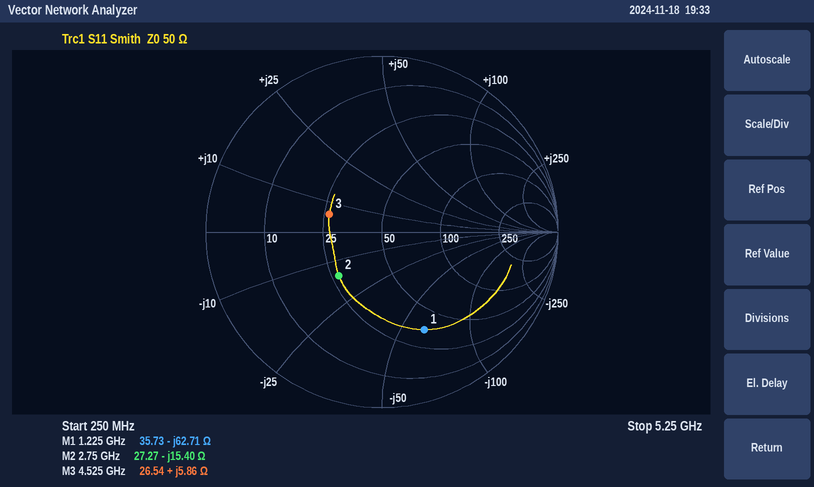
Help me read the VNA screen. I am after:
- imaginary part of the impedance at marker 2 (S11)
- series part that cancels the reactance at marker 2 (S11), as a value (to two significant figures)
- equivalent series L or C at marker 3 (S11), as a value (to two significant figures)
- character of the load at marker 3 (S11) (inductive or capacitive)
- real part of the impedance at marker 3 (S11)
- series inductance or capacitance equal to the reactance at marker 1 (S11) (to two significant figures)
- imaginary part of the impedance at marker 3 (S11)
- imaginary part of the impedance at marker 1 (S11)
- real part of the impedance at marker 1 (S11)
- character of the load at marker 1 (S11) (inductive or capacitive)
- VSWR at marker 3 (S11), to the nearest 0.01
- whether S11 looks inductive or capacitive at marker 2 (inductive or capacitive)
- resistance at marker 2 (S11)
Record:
-15.40 Ω
890 pH
210 pH
inductive
26.54 Ω
2.1 pF
+5.86 Ω
-62.71 Ω
35.73 Ω
capacitive
1.92
capacitive
27.27 Ω
